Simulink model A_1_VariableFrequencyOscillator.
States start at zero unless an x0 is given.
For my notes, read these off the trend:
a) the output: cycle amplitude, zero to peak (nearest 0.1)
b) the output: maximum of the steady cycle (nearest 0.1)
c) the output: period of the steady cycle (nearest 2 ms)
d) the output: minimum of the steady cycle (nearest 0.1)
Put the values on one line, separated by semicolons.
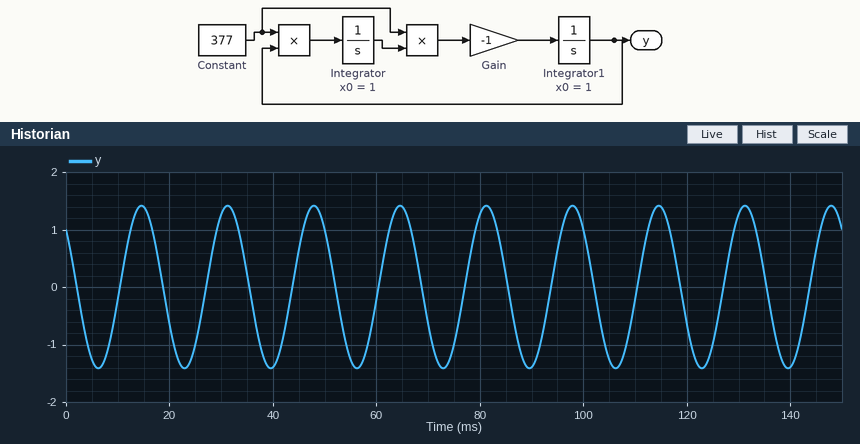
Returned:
1.4; 1.4; 16 ms; -1.4
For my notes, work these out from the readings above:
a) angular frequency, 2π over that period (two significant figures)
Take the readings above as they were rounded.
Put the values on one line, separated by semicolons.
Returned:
0.39 rad/ms
